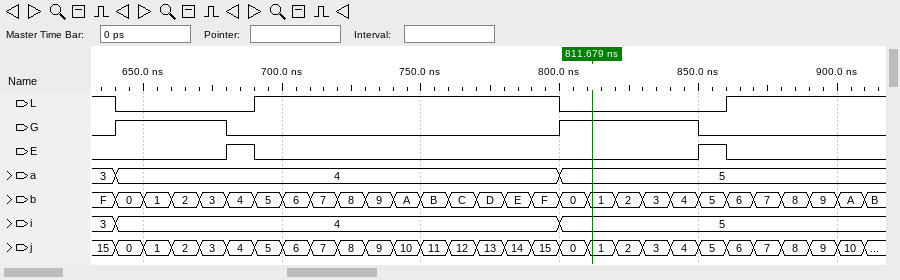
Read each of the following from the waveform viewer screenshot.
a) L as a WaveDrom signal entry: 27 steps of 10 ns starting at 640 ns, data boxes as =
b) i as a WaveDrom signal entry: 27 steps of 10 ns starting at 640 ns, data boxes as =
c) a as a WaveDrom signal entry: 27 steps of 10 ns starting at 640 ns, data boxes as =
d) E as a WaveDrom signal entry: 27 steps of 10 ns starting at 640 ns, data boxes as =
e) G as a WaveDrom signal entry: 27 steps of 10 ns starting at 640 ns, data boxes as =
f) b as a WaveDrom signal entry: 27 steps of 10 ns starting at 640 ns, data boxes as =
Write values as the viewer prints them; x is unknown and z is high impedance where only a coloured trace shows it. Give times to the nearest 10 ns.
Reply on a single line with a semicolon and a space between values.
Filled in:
{name: 'L', wave: '0....1..........0.....1....'}; {name: 'i', wave: '=...............=..........', data: '4 5'}; {name: 'a', wave: '=...............=..........', data: '4 5'}; {name: 'E', wave: '0...10...............10....'}; {name: 'G', wave: '1...0...........1....0.....'}; {name: 'b', wave: '===========================', data: '0 1 2 3 4 5 6 7 8 9 A B C D E F 0 1 2 3 4 5 6 7 8 9 A'}
